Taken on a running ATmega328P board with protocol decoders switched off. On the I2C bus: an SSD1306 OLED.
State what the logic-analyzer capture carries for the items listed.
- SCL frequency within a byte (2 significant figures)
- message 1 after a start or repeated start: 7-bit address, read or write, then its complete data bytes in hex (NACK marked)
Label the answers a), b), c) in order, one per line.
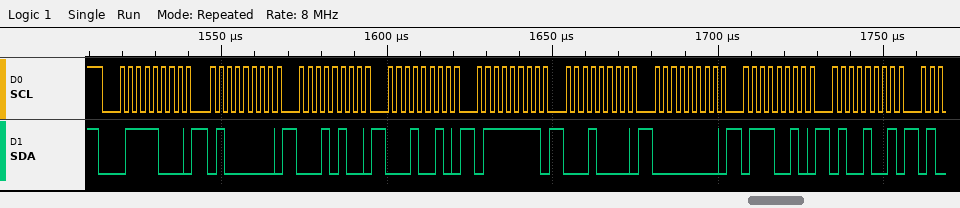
a) 400 kHz
b) 0x3C write: 40 14 12 7F 10 00 72 49
